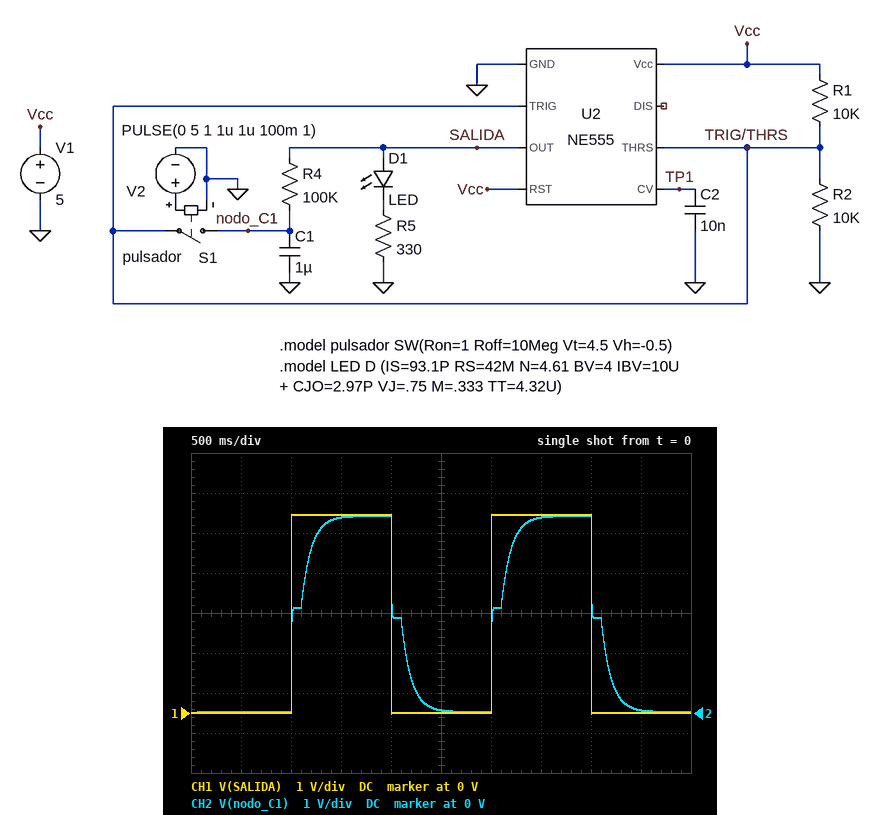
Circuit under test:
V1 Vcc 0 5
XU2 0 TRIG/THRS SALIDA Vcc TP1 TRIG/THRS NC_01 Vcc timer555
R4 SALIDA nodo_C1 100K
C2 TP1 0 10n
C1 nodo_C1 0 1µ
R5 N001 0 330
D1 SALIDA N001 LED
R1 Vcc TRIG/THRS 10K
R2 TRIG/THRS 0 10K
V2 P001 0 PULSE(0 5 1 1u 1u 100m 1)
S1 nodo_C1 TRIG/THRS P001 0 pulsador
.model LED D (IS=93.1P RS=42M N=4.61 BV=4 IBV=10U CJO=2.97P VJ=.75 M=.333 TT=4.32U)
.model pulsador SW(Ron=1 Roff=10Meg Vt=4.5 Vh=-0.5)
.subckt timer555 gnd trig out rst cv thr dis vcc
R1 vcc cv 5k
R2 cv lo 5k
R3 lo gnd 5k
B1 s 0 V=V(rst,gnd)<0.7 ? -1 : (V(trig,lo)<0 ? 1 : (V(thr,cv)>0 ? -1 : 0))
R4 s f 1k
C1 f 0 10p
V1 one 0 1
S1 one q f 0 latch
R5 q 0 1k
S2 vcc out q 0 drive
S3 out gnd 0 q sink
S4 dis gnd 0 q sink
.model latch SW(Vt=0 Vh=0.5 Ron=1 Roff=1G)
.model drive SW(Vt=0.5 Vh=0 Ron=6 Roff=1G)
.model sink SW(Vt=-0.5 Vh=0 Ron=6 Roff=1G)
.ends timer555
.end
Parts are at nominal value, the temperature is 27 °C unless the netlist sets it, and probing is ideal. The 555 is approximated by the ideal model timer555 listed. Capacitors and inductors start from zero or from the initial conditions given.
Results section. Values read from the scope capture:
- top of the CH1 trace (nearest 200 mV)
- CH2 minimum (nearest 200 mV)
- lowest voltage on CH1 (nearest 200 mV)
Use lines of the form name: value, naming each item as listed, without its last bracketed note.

top of the CH1 trace: 5.0 V
CH2 minimum: 0 V
lowest voltage on CH1: 0 V
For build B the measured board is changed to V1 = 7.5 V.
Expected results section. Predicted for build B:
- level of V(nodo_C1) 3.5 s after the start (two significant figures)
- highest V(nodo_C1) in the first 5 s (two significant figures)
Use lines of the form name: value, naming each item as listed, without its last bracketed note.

level of V(nodo_C1) 3.5 s after the start: 7.3 V
highest V(nodo_C1) in the first 5 s: 7.4 V
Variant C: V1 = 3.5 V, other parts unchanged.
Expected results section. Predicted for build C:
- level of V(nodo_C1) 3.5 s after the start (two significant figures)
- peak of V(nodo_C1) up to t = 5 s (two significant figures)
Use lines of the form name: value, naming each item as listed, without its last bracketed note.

level of V(nodo_C1) 3.5 s after the start: 3.4 V
peak of V(nodo_C1) up to t = 5 s: 3.5 V
